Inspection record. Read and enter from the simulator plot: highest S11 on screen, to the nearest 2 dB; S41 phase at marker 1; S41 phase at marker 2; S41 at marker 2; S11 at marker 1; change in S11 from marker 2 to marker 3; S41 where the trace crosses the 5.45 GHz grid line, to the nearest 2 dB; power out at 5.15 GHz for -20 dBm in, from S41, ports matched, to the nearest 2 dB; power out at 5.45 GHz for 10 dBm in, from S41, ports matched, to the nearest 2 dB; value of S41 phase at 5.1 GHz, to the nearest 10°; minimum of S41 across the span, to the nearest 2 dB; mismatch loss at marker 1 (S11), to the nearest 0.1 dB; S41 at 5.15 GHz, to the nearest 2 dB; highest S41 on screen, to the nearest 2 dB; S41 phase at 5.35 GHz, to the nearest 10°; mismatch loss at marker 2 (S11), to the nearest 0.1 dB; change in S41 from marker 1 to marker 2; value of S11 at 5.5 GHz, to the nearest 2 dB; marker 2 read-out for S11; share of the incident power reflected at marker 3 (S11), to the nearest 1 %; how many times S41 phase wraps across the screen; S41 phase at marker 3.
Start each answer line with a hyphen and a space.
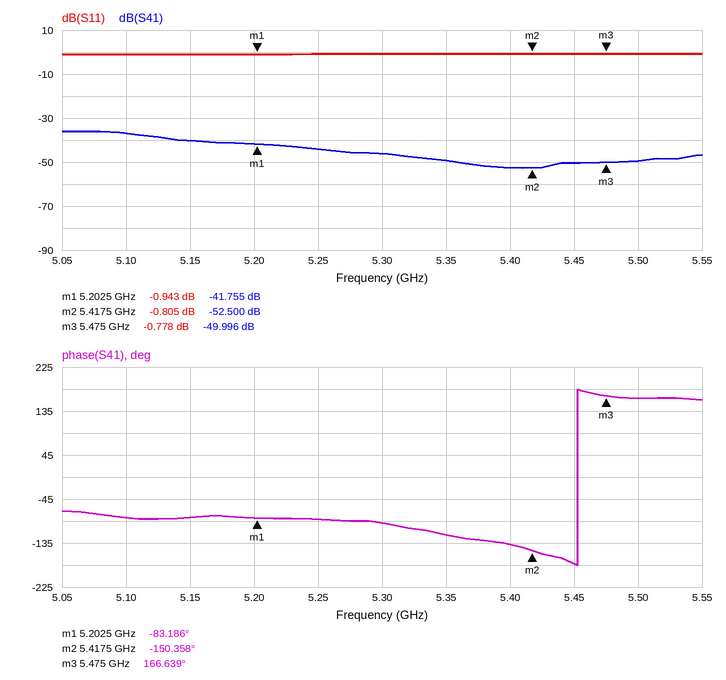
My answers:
- 0 dB
- -83.186°
- -150.358°
- -52.500 dB
- -0.943 dB
- 0.027 dB
- -50 dB
- -60 dBm
- -40 dBm
- -80°
- -52 dB
- 7.1 dB
- -40 dB
- -36 dB
- -120°
- 7.7 dB
- -10.745 dB
- 0 dB
- -0.805 dB
- 84 %
- 1
- 166.639°
